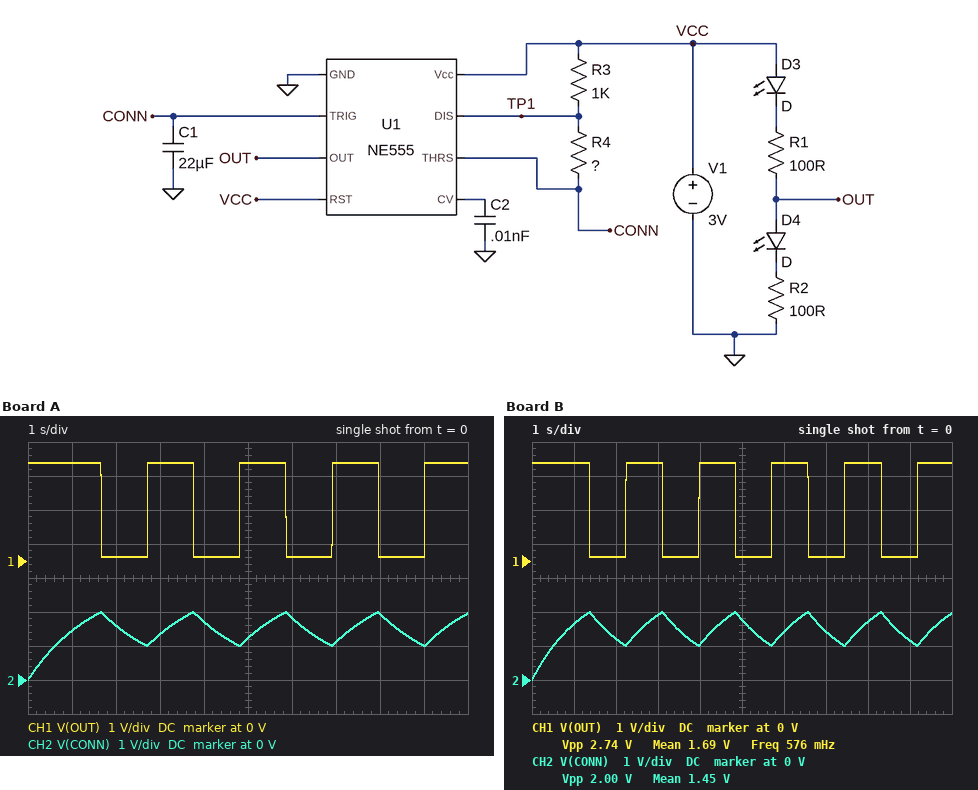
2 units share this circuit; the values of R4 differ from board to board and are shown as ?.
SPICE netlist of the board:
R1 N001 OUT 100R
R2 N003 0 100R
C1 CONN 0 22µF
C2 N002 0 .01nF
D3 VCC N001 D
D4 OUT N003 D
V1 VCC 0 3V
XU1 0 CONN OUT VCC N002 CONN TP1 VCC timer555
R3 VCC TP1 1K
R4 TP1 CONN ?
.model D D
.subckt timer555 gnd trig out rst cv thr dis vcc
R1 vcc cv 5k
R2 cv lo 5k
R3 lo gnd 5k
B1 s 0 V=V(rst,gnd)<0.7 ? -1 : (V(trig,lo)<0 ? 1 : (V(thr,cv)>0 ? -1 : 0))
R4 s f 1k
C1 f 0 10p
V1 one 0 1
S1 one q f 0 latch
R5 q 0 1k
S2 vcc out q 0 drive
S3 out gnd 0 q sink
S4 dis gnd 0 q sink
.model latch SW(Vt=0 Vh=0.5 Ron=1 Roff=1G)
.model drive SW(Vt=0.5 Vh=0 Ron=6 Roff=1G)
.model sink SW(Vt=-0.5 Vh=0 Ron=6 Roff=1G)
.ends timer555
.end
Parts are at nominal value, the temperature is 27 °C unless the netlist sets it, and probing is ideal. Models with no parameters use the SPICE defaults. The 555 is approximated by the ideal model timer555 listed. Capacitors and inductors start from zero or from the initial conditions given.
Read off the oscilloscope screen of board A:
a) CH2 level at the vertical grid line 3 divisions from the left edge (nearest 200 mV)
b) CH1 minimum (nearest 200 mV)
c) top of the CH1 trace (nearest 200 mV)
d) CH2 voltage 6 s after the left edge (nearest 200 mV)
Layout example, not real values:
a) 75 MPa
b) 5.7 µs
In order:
a) 1.4 V
b) 200 mV
c) 2.8 V
d) 1.8 V
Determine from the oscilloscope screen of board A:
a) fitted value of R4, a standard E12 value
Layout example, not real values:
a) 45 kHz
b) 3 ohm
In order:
a) 68 kΩ
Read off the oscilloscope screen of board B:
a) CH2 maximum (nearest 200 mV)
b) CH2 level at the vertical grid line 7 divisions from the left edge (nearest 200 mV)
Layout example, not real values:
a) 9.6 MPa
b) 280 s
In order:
a) 2.0 V
b) 1.4 V
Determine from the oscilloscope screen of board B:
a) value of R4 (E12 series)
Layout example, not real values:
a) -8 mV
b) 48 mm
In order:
a) 56 kΩ
